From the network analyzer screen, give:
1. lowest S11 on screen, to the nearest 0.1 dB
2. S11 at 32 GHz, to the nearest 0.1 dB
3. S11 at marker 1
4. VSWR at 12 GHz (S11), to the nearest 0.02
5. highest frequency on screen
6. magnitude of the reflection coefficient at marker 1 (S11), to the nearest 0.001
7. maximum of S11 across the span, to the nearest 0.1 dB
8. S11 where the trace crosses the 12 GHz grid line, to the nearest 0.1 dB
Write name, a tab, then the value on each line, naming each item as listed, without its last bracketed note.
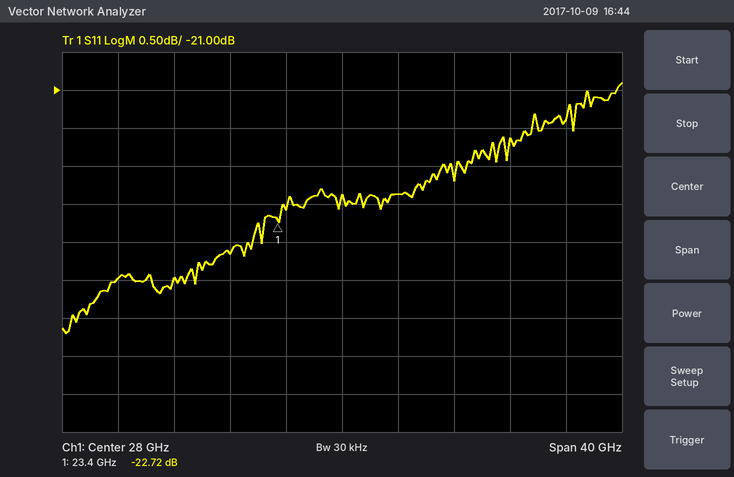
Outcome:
lowest S11 on screen, to the nearest 0.1 dB	-24.2 dB
S11 at 32 GHz, to the nearest 0.1 dB	-22.4 dB
S11 at marker 1	-22.72 dB
VSWR at 12 GHz (S11), to the nearest 0.02	1.14
highest frequency on screen	48 GHz
magnitude of the reflection coefficient at marker 1 (S11), to the nearest 0.001	0.073
maximum of S11 across the span, to the nearest 0.1 dB	-20.9 dB
S11 where the trace crosses the 12 GHz grid line, to the nearest 0.1 dB	-23.5 dB
